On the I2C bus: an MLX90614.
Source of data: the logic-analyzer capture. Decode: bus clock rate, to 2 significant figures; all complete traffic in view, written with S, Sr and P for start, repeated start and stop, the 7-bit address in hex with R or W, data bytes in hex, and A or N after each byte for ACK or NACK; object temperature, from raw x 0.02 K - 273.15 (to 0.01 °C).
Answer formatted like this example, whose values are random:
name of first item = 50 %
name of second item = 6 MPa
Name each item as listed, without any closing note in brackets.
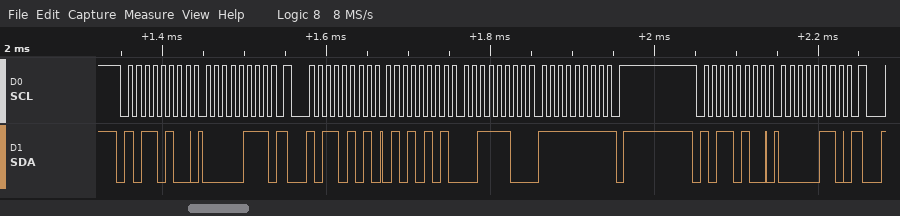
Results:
bus clock rate, to 2 significant figures = 100 kHz
all complete traffic in view, written with S, Sr and P for start, repeated start and stop, the 7-bit address in hex with R or W, data bytes in hex, and A or N after each byte for ACK or NACK = S 5AW A 07 A Sr 5AR A 55 A 3C A FF N P S 5AW A 06 A
object temperature, from raw x 0.02 K - 273.15 = 35.75 °C
